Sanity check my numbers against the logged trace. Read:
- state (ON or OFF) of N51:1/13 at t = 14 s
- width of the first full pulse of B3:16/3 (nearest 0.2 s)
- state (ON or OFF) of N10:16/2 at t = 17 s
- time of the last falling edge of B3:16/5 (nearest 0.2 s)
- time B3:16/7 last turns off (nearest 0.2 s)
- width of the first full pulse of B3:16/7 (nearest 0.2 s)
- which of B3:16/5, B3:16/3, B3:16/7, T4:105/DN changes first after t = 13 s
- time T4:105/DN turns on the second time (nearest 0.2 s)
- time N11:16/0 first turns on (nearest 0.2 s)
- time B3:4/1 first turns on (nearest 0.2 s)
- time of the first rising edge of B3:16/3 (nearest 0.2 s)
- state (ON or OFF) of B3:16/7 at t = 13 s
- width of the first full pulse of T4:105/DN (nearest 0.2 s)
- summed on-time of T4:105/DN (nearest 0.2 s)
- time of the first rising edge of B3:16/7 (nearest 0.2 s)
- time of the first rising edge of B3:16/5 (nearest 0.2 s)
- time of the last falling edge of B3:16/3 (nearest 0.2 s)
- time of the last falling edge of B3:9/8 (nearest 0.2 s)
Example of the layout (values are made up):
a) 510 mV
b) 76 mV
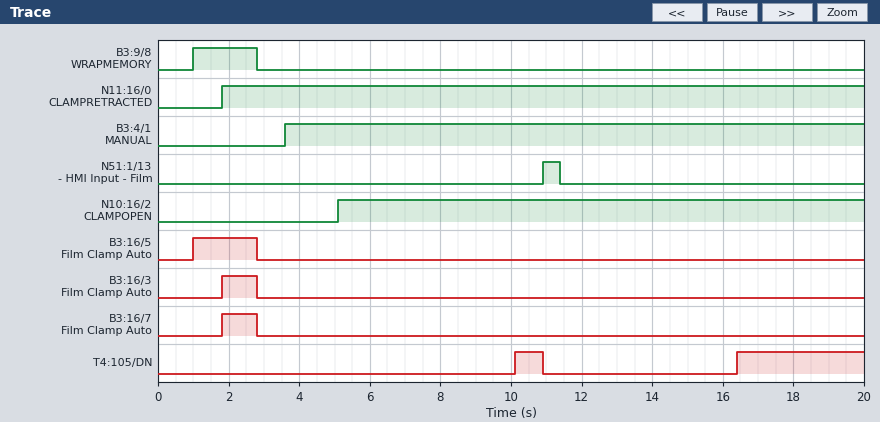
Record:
a) OFF
b) 1.0 s
c) ON
d) 2.8 s
e) 2.8 s
f) 1.0 s
g) T4:105/DN
h) 16.4 s
i) 1.8 s
j) 3.6 s
k) 1.8 s
l) OFF
m) 0.8 s
n) 4.4 s
o) 1.8 s
p) 1.0 s
q) 2.8 s
r) 2.8 s
